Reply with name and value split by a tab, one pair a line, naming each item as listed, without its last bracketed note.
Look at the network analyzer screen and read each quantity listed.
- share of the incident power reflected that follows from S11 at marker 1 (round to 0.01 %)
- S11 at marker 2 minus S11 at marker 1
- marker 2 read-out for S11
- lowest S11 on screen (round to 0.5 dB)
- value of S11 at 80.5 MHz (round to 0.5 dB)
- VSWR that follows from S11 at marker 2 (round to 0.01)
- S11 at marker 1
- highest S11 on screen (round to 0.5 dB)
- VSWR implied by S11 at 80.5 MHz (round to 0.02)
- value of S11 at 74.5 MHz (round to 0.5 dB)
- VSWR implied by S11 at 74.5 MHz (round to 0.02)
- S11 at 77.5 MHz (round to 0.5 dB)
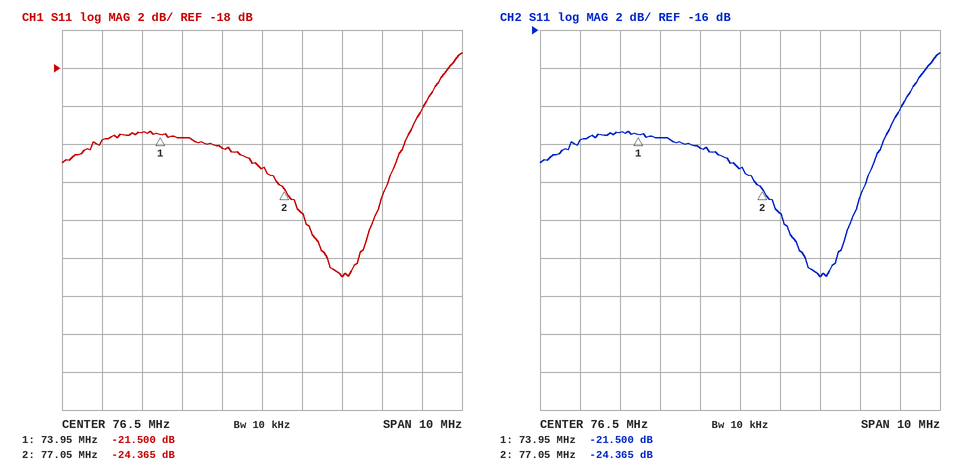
share of the incident power reflected that follows from S11 at marker 1	0.71 %
S11 at marker 2 minus S11 at marker 1	-2.865 dB
marker 2 read-out for S11	-24.365 dB
lowest S11 on screen	-29.0 dB
value of S11 at 80.5 MHz	-20.0 dB
VSWR that follows from S11 at marker 2	1.13
S11 at marker 1	-21.500 dB
highest S11 on screen	-17.0 dB
VSWR implied by S11 at 80.5 MHz	1.22
value of S11 at 74.5 MHz	-21.5 dB
VSWR implied by S11 at 74.5 MHz	1.18
S11 at 77.5 MHz	-25.5 dB
